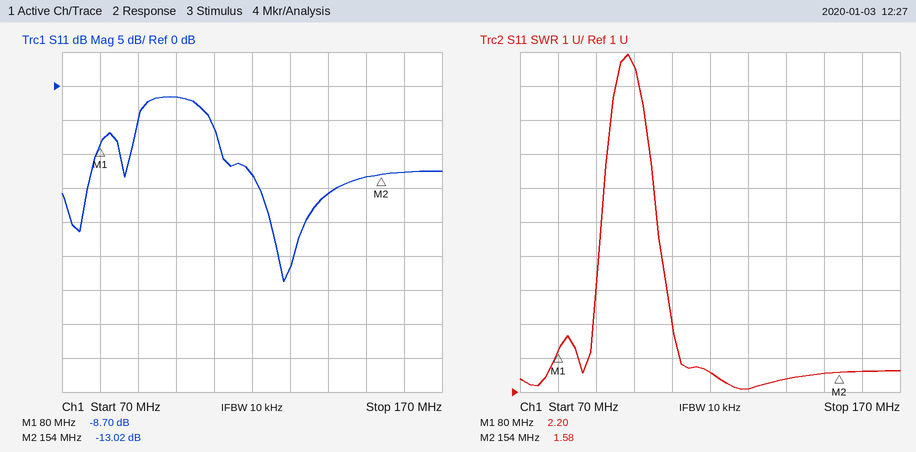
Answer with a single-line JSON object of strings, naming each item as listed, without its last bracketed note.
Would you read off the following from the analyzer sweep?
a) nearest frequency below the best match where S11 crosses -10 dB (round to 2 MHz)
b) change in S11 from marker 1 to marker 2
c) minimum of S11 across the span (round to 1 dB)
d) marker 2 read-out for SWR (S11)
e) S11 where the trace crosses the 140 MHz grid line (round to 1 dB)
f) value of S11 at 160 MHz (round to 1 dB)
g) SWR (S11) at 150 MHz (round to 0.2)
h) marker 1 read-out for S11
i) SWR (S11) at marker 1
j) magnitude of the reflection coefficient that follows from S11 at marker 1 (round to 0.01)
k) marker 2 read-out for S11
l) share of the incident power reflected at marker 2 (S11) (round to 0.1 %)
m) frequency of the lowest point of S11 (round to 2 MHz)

{"nearest frequency below the best match where S11 crosses -10 dB": "112 MHz", "change in S11 from marker 1 to marker 2": "-4.32 dB", "minimum of S11 across the span": "-29 dB", "marker 2 read-out for SWR": "1.58", "S11 where the trace crosses the 140 MHz grid line": "-16 dB", "value of S11 at 160 MHz": "-13 dB", "SWR (S11) at 150 MHz": "1.6", "marker 1 read-out for S11": "-8.70 dB", "SWR (S11) at marker 1": "2.20", "magnitude of the reflection coefficient that follows from S11 at marker 1": "0.37", "marker 2 read-out for S11": "-13.02 dB", "share of the incident power reflected at marker 2 (S11)": "5.0 %", "frequency of the lowest point of S11": "128 MHz"}
